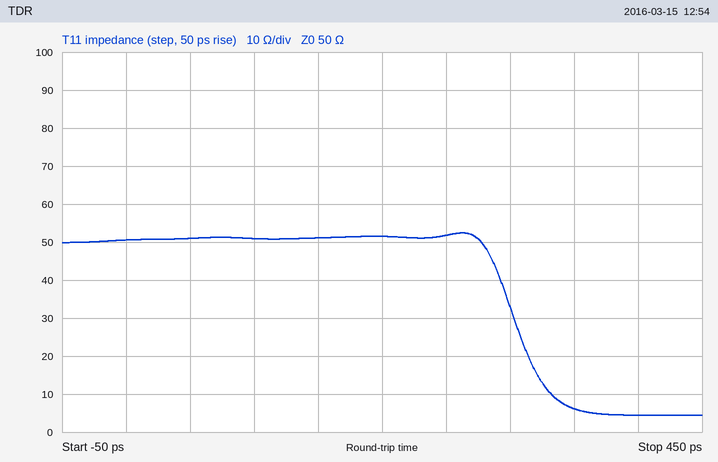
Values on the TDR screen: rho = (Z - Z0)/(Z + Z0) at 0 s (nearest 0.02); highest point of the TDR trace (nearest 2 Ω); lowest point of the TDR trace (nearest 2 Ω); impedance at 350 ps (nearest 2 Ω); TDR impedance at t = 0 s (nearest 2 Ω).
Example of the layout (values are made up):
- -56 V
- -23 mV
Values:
- 0.00
- 52 Ω
- 4 Ω
- 6 Ω
- 50 Ω
